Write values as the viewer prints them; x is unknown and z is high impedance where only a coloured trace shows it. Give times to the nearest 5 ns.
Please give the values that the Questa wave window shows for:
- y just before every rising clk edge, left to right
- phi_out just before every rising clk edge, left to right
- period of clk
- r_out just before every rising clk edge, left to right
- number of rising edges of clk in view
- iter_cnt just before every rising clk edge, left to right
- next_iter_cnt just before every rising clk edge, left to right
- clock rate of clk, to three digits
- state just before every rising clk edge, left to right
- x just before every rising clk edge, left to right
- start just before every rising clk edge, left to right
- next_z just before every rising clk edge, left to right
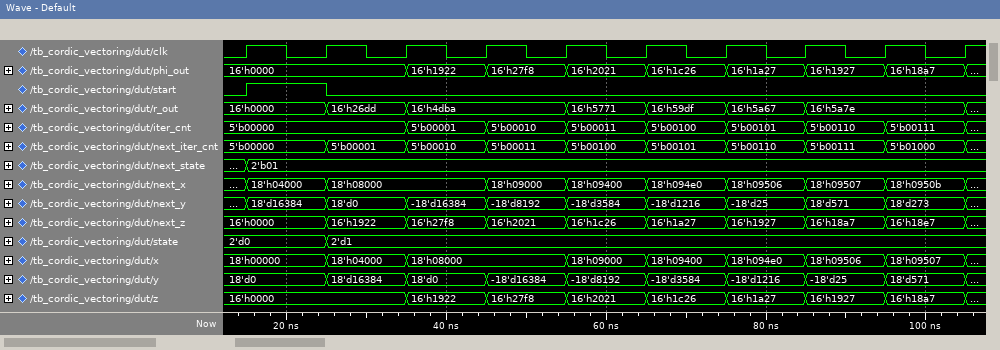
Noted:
18'd0, 18'd0, 18'd16384, 18'd0, -18'd16384, -18'd8192, -18'd3584, -18'd1216, -18'd25, 18'd571
16'h0000, 16'h0000, 16'h0000, 16'h1922, 16'h27f8, 16'h2021, 16'h1c26, 16'h1a27, 16'h1927, 16'h18a7
10 ns
16'h0000, 16'h0000, 16'h26dd, 16'h4dba, 16'h4dba, 16'h5771, 16'h59df, 16'h5a67, 16'h5a7e, 16'h5a7e
10
5'b00000, 5'b00000, 5'b00000, 5'b00001, 5'b00010, 5'b00011, 5'b00100, 5'b00101, 5'b00110, 5'b00111
5'b00000, 5'b00000, 5'b00001, 5'b00010, 5'b00011, 5'b00100, 5'b00101, 5'b00110, 5'b00111, 5'b01000
100 MHz
2'd0, 2'd0, 2'd1, 2'd1, 2'd1, 2'd1, 2'd1, 2'd1, 2'd1, 2'd1
18'h00000, 18'h00000, 18'h04000, 18'h08000, 18'h08000, 18'h09000, 18'h09400, 18'h094e0, 18'h09506, 18'h09507
0 1 0 0 0 0 0 0 0 0
16'h0000, 16'h0000, 16'h1922, 16'h27f8, 16'h2021, 16'h1c26, 16'h1a27, 16'h1927, 16'h18a7, 16'h18e7
